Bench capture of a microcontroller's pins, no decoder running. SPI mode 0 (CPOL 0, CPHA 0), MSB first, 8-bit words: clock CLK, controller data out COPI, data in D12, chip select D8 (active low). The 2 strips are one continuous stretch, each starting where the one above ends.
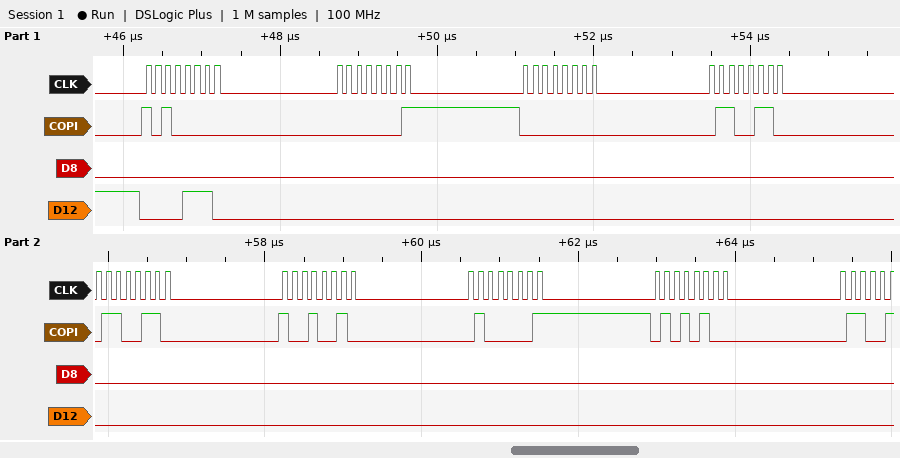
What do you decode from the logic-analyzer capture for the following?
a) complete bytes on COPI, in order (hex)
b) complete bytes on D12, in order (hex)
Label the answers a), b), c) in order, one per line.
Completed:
a) A0 01 00 66 66 92 41 54
b) 0E 00 00 00 00 00 00 00
